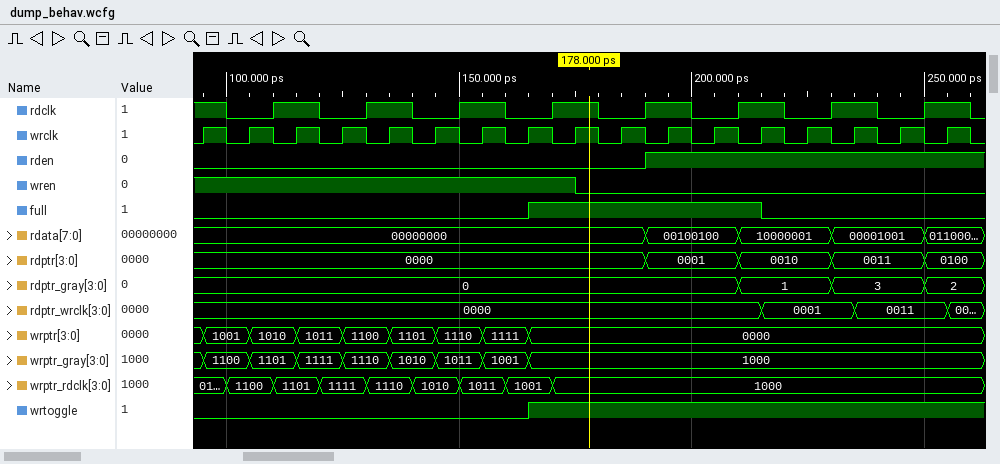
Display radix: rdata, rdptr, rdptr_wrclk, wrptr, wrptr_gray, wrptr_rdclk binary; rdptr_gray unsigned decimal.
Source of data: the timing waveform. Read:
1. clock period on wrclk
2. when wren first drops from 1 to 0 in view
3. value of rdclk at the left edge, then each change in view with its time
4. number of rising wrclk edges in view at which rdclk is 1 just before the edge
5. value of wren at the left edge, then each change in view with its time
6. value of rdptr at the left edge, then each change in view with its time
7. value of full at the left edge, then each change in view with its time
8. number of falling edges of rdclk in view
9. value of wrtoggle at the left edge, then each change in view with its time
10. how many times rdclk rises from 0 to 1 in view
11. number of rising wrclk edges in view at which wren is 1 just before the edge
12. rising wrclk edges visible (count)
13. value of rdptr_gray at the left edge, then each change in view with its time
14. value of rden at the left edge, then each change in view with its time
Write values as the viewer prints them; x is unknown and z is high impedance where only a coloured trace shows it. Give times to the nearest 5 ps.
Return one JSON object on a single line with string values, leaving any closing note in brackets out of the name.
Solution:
{"clock period on wrclk": "10 ps", "when wren first drops from 1 to 0 in view": "175 ps", "value of rdclk at the left edge, then each change in view with its time": "1, 0 at 100 ps, 1 at 110 ps, 0 at 120 ps, 1 at 130 ps, 0 at 140 ps, 1 at 150 ps, 0 at 160 ps, 1 at 170 ps, 0 at 180 ps, 1 at 190 ps, 0 at 200 ps, 1 at 210 ps, 0 at 220 ps, 1 at 230 ps, 0 at 240 ps, 1 at 250 ps, 0 at 260 ps", "number of rising wrclk edges in view at which rdclk is 1 just before the edge": "9", "value of wren at the left edge, then each change in view with its time": "1, 0 at 175 ps", "value of rdptr at the left edge, then each change in view with its time": "0000, 0001 at 190 ps, 0010 at 210 ps, 0011 at 230 ps, 0100 at 250 ps", "value of full at the left edge, then each change in view with its time": "0, 1 at 165 ps, 0 at 215 ps", "number of falling edges of rdclk in view": "9", "value of wrtoggle at the left edge, then each change in view with its time": "0, 1 at 165 ps", "how many times rdclk rises from 0 to 1 in view": "8", "number of rising wrclk edges in view at which wren is 1 just before the edge": "9", "rising wrclk edges visible": "17", "value of rdptr_gray at the left edge, then each change in view with its time": "0, 1 at 210 ps, 3 at 230 ps, 2 at 250 ps", "value of rden at the left edge, then each change in view with its time": "0, 1 at 190 ps"}
